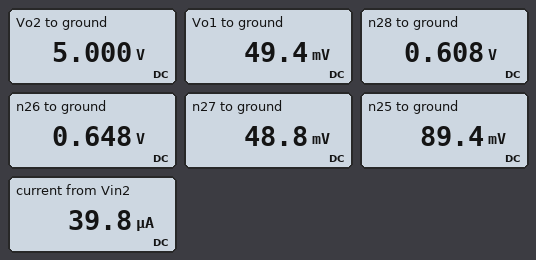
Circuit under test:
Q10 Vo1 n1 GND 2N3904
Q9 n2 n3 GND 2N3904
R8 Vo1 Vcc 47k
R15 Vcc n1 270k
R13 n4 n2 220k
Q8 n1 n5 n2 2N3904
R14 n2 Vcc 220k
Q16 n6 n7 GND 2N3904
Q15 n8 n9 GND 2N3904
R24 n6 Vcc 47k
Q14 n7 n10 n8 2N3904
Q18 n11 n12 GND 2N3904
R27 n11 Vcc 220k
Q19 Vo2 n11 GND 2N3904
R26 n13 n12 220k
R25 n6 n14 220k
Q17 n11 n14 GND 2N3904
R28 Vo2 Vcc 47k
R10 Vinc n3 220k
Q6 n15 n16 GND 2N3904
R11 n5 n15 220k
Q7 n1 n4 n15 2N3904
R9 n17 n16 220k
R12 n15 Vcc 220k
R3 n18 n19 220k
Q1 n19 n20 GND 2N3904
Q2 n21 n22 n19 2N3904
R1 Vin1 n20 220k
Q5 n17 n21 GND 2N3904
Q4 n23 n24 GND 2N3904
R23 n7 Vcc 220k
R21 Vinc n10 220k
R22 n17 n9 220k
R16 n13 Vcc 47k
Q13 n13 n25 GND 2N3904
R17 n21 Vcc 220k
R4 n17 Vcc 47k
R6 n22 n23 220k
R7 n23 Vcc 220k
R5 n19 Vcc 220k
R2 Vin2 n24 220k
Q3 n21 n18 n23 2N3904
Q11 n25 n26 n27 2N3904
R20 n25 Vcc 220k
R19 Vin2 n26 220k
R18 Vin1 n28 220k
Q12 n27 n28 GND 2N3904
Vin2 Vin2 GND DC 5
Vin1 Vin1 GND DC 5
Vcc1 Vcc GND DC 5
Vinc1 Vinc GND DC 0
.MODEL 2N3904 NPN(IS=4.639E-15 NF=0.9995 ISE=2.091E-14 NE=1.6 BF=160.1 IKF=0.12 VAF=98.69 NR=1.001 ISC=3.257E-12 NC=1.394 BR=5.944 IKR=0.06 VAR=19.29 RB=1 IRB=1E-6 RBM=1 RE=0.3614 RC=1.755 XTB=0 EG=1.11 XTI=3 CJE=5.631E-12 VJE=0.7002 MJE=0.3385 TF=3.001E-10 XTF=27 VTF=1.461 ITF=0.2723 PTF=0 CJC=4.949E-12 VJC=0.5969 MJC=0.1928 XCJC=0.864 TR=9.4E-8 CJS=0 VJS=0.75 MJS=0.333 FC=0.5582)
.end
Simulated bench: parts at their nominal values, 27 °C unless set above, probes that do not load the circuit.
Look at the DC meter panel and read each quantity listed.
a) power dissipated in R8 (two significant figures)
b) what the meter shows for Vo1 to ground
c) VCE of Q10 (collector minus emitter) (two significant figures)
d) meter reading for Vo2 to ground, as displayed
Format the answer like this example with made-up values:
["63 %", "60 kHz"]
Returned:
["520 µW", "49.4 mV", "49 mV", "5.000 V"]
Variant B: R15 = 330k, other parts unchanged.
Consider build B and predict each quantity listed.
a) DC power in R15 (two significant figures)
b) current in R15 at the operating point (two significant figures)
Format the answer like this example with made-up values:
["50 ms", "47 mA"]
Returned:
["58 µW", "13 µA"]
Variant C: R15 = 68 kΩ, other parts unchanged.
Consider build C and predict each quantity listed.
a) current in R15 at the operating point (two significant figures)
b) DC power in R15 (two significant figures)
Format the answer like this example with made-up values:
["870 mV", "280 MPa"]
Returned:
["64 µA", "280 µW"]
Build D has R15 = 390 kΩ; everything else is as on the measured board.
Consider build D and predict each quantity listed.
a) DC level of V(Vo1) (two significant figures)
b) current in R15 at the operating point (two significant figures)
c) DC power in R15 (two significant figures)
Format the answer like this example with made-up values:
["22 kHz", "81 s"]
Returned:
["53 mV", "11 µA", "49 µW"]
